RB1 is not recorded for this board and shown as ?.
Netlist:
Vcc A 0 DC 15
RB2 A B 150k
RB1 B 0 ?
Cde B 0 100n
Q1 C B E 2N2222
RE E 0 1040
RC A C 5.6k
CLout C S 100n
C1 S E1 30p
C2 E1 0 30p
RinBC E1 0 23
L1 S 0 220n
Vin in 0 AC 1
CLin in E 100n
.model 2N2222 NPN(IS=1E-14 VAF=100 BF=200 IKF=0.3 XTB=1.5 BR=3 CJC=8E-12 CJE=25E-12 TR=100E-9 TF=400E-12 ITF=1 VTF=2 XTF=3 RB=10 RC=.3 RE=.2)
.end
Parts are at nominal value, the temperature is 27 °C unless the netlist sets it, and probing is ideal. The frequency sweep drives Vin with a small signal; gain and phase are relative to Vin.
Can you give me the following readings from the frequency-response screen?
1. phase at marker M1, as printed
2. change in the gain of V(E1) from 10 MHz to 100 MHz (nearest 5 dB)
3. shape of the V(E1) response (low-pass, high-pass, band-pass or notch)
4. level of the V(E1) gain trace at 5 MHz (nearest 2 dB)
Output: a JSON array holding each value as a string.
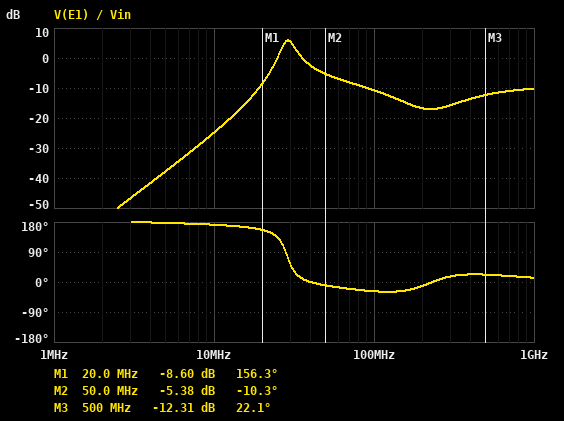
["156.3 deg", "15 dB", "band-pass", "-38 dB"]
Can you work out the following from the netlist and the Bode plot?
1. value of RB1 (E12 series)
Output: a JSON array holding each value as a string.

["47 kΩ"]
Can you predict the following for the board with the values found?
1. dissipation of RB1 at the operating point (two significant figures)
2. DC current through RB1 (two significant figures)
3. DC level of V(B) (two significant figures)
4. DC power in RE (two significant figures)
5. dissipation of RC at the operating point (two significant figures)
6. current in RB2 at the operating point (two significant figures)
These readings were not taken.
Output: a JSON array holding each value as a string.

["190 µW", "64 µA", "3.0 V", "5.3 mW", "28 mW", "80 µA"]
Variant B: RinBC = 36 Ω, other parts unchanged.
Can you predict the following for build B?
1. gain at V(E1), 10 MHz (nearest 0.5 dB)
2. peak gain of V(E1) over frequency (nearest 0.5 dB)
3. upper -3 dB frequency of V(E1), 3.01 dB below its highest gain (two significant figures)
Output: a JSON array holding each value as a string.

["-21.0 dB", "9.0 dB", "33 MHz"]
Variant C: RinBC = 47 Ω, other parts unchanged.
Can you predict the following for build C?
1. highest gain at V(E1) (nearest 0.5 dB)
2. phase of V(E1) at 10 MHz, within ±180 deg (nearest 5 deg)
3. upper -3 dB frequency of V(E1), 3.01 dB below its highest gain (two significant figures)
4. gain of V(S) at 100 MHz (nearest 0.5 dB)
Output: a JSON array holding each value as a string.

["10.5 dB", "165 deg", "33 MHz", "-0.5 dB"]
